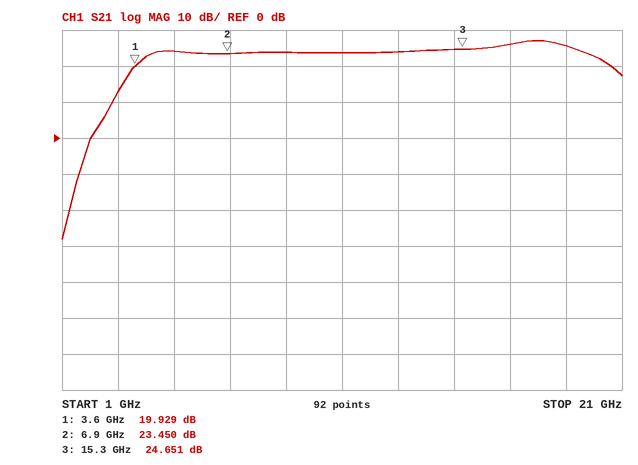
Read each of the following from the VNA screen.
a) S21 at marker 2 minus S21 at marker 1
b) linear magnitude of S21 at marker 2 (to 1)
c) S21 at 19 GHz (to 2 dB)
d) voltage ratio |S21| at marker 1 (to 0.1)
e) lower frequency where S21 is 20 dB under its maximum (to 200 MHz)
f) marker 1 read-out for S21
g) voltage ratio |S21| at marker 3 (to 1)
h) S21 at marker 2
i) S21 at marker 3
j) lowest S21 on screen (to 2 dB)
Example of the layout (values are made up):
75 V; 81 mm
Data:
3.521 dB; 15; 26 dB; 9.9; 2.6 GHz; 19.929 dB; 17; 23.450 dB; 24.651 dB; -28 dB
